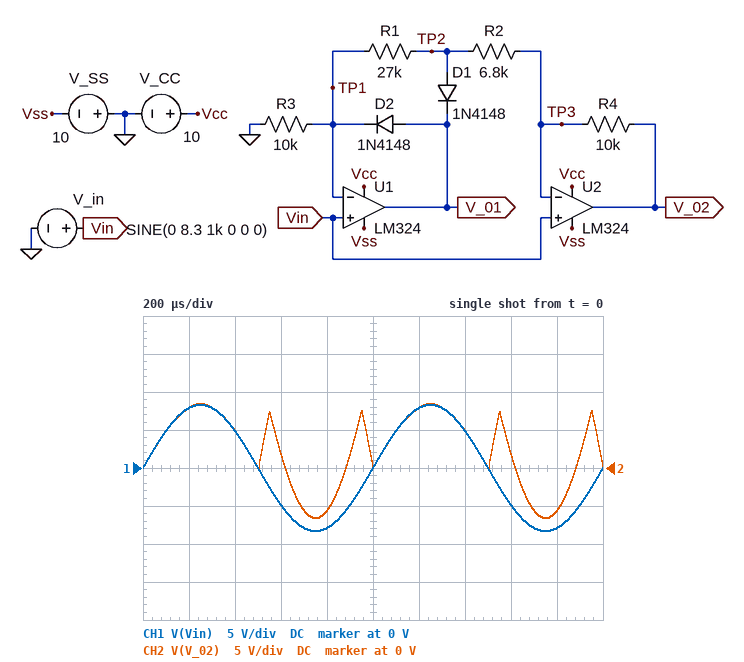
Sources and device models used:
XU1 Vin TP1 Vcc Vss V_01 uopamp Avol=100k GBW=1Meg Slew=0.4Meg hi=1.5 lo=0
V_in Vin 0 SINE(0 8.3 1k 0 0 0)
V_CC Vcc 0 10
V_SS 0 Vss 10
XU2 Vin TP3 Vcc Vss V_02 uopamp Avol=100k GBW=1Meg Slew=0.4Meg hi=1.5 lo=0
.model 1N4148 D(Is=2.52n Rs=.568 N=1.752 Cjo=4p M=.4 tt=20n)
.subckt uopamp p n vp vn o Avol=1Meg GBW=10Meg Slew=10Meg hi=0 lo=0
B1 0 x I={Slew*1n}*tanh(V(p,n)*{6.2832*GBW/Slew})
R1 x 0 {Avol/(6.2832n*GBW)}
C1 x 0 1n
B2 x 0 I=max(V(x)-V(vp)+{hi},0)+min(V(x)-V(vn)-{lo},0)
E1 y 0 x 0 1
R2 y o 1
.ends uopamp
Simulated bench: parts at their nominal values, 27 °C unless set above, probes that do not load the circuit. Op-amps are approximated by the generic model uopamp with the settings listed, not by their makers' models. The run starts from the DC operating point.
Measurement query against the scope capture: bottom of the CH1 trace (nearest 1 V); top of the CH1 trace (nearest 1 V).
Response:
-8 V
8 V
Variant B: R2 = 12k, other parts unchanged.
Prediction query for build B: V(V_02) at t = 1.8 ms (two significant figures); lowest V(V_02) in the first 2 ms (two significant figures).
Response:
-6.6 V
-7.3 V
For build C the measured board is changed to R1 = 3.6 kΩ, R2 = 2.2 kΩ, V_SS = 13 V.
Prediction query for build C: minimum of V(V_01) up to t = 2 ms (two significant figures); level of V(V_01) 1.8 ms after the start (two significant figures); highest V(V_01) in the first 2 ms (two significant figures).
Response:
-12 V
-11 V
8.5 V
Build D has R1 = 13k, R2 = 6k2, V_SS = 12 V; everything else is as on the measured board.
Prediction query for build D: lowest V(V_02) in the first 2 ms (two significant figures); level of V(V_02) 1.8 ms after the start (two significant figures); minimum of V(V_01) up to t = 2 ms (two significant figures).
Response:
-3.3 V
-2.2 V
-12 V
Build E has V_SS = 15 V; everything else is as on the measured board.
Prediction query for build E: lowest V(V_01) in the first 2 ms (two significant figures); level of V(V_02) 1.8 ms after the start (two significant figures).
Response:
-15 V
1.7 V
